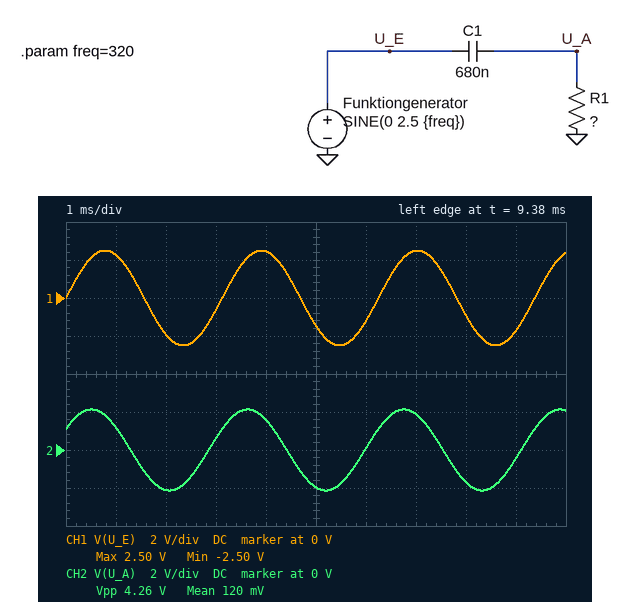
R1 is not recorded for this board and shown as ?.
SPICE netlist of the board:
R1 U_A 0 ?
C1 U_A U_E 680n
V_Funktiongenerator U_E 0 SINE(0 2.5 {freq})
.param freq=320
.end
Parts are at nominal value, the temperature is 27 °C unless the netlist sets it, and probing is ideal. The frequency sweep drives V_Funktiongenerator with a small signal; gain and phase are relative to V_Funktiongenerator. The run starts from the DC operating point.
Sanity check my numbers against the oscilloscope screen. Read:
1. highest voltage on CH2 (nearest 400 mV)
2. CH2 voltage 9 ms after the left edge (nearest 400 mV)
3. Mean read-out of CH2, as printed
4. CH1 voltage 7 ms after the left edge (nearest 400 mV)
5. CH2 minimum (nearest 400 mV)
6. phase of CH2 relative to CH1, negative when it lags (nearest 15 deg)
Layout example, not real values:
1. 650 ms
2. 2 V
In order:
1. 2.0 V
2. -400 mV
3. 120 mV
4. 2.4 V
5. -2.0 V
6. 30 deg
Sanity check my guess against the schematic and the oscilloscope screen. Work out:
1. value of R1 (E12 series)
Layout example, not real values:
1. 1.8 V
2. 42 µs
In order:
1. 1.2 kΩ
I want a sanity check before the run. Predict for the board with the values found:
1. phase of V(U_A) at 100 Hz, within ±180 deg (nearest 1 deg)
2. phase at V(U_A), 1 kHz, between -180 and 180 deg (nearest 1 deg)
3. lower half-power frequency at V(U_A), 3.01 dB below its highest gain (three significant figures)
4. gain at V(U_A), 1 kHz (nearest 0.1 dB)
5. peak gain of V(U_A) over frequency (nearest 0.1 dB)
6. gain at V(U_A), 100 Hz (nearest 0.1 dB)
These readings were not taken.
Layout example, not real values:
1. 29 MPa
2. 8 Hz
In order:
1. 63 deg
2. 11 deg
3. 195 Hz
4. -0.2 dB
5. 0 dB
6. -6.8 dB
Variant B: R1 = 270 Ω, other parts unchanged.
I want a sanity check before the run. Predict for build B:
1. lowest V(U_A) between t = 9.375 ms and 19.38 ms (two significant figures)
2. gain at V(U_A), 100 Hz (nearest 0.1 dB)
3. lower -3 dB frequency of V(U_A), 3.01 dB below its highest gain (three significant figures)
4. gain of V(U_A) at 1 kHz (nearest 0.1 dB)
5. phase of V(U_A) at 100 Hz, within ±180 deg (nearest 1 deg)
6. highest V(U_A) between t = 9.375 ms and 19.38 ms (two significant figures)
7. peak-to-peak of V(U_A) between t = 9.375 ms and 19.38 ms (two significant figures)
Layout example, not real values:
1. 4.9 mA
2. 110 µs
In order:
1. -870 mV
2. -18.8 dB
3. 867 Hz
4. -2.4 dB
5. 83 deg
6. 870 mV
7. 1.7 V
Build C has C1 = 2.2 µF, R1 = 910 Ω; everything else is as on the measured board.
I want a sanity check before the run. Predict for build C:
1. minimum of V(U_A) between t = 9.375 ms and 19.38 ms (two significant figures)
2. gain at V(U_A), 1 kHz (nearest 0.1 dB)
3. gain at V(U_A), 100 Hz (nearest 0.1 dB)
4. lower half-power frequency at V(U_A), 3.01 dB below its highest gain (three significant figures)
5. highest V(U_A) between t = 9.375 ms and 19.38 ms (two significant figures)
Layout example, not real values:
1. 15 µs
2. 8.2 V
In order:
1. -2.4 V
2. 0 dB
3. -2.1 dB
4. 79.5 Hz
5. 2.4 V
